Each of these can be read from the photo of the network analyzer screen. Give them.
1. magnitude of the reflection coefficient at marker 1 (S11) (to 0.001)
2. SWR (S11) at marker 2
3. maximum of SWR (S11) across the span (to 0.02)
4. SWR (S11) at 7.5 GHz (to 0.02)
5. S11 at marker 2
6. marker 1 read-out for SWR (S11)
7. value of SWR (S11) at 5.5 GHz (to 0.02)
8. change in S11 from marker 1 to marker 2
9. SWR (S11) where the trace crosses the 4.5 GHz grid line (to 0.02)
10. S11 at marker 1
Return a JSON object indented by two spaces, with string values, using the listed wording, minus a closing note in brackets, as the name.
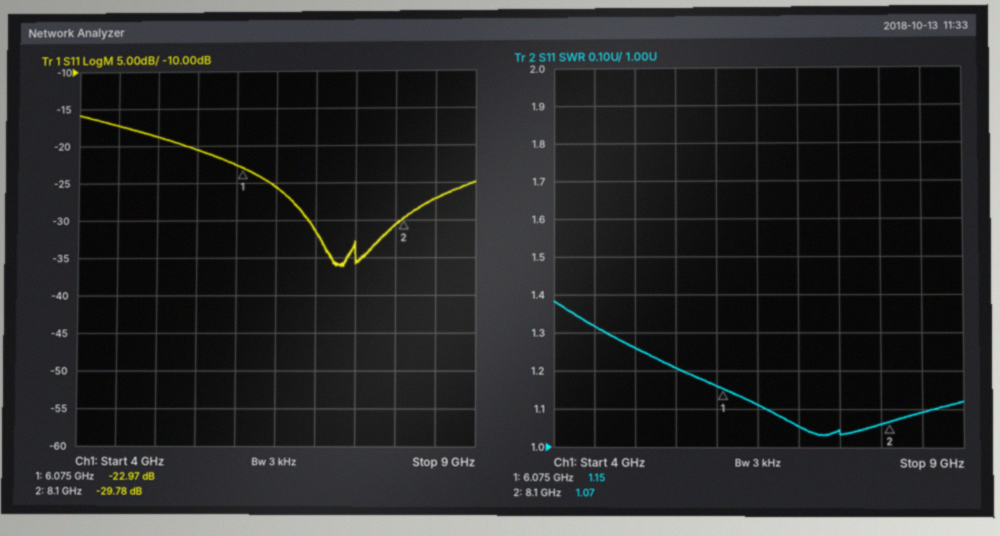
{
  "magnitude of the reflection coefficient at marker 1 (S11)": "0.071",
  "SWR (S11) at marker 2": "1.07",
  "maximum of SWR (S11) across the span": "1.38",
  "SWR (S11) at 7.5 GHz": "1.04",
  "S11 at marker 2": "-29.78 dB",
  "marker 1 read-out for SWR": "1.15",
  "value of SWR (S11) at 5.5 GHz": "1.20",
  "change in S11 from marker 1 to marker 2": "-6.81 dB",
  "SWR (S11) where the trace crosses the 4.5 GHz grid line": "1.32",
  "S11 at marker 1": "-22.97 dB"
}
